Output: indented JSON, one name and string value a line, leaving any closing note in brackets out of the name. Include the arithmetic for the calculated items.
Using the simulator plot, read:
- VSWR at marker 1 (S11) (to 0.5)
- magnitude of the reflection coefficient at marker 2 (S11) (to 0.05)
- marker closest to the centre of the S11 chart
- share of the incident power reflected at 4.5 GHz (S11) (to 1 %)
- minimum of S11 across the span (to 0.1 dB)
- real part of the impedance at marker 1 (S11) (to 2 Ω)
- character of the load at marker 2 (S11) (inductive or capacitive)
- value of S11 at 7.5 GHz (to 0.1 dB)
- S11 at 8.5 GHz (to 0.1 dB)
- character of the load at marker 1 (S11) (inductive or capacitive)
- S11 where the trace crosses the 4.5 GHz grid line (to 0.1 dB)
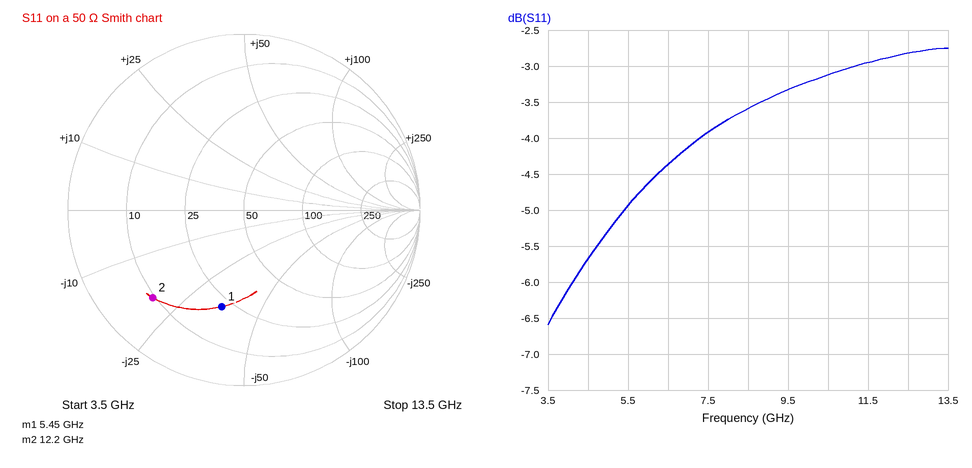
{
  "VSWR at marker 1 (S11)": "3.5",
  "magnitude of the reflection coefficient at marker 2 (S11)": "0.70",
  "marker closest to the centre of the S11 chart": "marker 1",
  "share of the incident power reflected at 4.5 GHz (S11)": "10^(-5.7/10) ≈ 27 %",
  "minimum of S11 across the span": "-6.6 dB",
  "real part of the impedance at marker 1 (S11)": "22 Ω",
  "character of the load at marker 2 (S11)": "capacitive",
  "value of S11 at 7.5 GHz": "-3.9 dB",
  "S11 at 8.5 GHz": "-3.6 dB",
  "character of the load at marker 1 (S11)": "capacitive",
  "S11 where the trace crosses the 4.5 GHz grid line": "-5.7 dB"
}
